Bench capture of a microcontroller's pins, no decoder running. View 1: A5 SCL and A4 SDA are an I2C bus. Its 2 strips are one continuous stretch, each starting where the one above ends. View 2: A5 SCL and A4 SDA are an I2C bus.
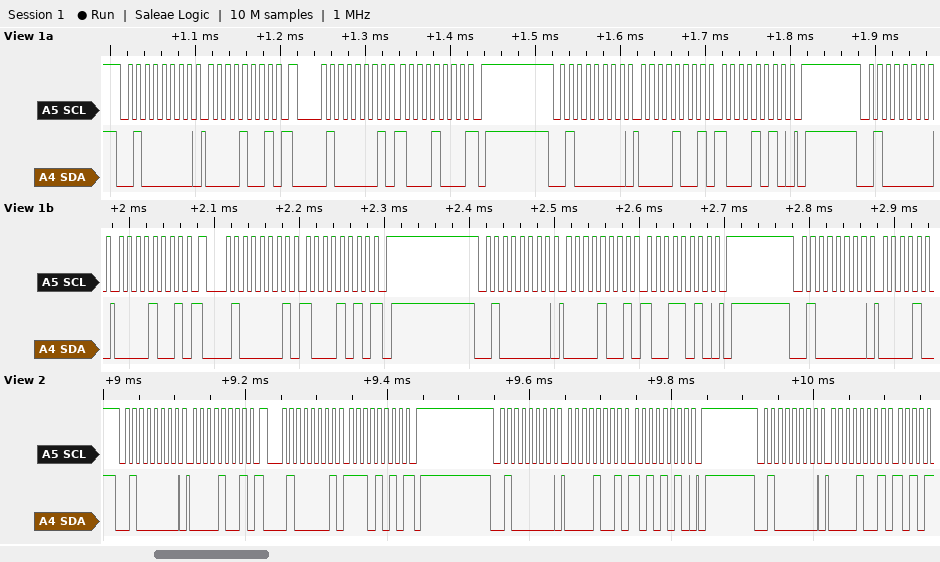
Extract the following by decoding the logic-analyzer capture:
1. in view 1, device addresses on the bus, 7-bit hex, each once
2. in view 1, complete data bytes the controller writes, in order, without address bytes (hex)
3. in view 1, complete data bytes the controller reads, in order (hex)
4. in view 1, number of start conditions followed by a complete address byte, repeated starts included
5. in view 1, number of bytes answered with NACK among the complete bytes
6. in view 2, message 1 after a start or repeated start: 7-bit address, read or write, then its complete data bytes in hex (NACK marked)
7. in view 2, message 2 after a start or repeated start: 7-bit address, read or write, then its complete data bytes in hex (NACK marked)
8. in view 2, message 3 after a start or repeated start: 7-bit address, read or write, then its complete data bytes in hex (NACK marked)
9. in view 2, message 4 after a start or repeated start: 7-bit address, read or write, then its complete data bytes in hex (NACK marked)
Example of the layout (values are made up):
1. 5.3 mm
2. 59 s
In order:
1. 0x20
2. 09 09 8A 09 09 9A
3. 88 8A
4. 7
5. 2
6. 0x20 write: 09
7. 0x20 read: EA NACK
8. 0x20 write: 09 AA
9. 0x20 write: 09
